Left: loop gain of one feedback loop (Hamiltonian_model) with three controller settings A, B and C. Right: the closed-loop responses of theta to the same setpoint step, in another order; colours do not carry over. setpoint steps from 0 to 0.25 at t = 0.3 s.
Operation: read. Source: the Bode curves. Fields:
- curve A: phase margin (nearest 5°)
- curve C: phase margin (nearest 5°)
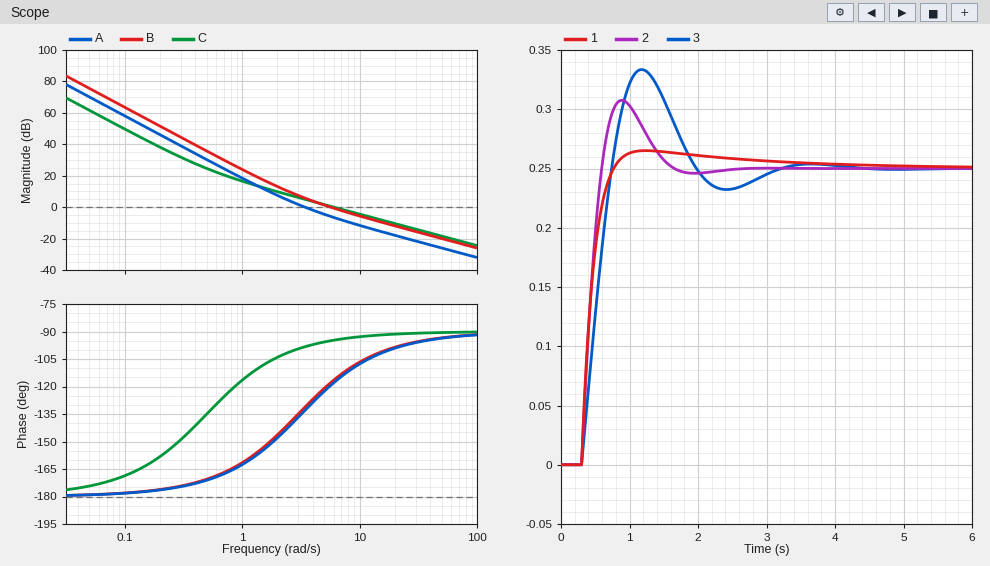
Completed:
45°
85°
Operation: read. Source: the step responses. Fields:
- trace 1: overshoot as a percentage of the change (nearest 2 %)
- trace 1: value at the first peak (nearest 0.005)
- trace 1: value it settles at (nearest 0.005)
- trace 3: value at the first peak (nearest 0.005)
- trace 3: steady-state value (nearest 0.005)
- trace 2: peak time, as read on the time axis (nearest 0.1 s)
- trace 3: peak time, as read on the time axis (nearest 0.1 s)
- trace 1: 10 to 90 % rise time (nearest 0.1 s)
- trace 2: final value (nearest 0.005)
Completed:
6 %
0.265
0.250
0.335
0.250
0.9 s
1.2 s
0.3 s
0.250
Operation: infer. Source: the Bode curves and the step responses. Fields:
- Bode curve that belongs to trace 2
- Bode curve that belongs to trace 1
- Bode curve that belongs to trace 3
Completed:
B
C
A
